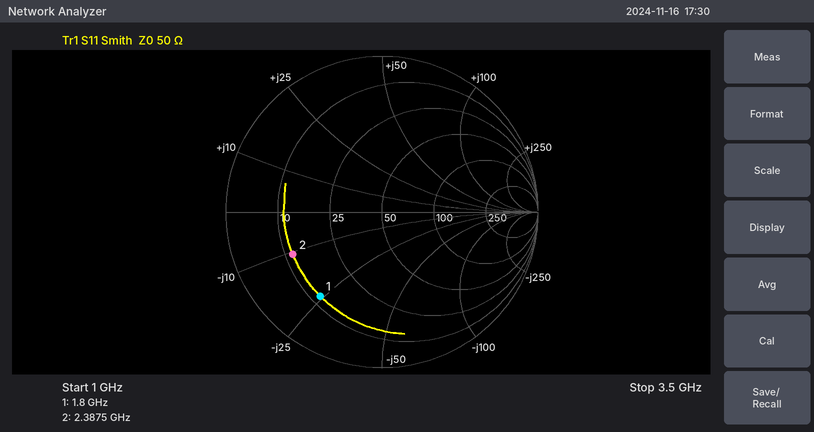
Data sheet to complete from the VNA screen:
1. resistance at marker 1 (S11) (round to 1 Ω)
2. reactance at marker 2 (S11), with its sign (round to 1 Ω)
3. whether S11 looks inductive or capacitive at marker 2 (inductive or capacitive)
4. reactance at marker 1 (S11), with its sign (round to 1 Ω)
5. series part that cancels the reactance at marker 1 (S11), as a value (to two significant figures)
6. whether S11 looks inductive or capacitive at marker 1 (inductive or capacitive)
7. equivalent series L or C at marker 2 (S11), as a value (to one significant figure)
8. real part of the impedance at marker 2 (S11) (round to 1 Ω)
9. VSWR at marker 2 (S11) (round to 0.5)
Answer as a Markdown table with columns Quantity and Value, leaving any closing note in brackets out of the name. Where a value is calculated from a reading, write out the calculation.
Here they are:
| Quantity | Value |
|---|---|
| resistance at marker 1 (S11) | 12 Ω |
| reactance at marker 2 (S11), with its sign | -11 Ω |
| whether S11 looks inductive or capacitive at marker 2 | capacitive |
| reactance at marker 1 (S11), with its sign | -24 Ω |
| series part that cancels the reactance at marker 1 (S11), as a value | L = 24 Ω/(2π × 1.8 GHz) ≈ 2.1 nH |
| whether S11 looks inductive or capacitive at marker 1 | capacitive |
| equivalent series L or C at marker 2 (S11), as a value | C = 1/(2π × 2.3875 GHz × 11 Ω) ≈ 6 pF |
| real part of the impedance at marker 2 (S11) | 12 Ω |
| VSWR at marker 2 (S11) | 4.5 |
